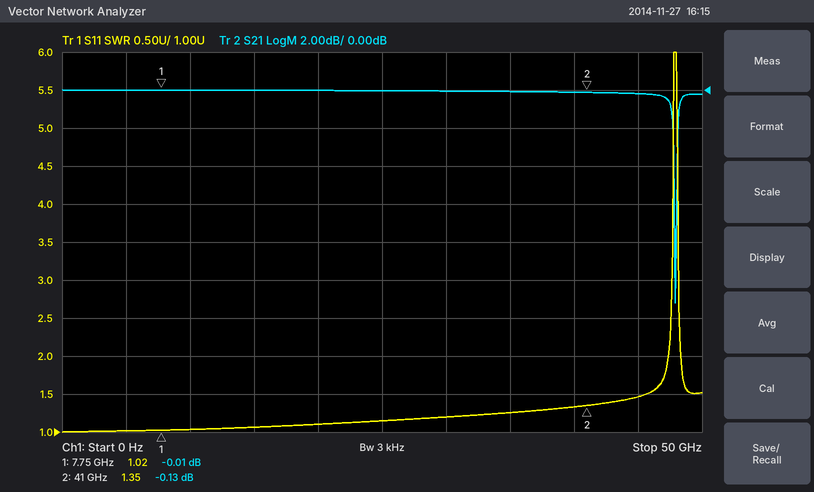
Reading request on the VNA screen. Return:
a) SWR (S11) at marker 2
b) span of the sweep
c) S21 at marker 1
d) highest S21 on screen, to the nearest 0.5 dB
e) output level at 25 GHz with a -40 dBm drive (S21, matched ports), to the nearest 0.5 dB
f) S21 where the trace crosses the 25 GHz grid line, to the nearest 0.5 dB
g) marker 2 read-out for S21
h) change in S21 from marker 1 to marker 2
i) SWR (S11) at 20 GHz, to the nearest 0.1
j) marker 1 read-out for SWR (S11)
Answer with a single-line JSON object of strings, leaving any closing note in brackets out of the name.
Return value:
{"SWR (S11) at marker 2": "1.35", "span of the sweep": "50 GHz", "S21 at marker 1": "-0.01 dB", "highest S21 on screen, to the nearest 0.5 dB": "0.0 dB", "output level at 25 GHz with a -40 dBm drive (S21, matched ports), to the nearest 0.5 dB": "-40.0 dBm", "S21 where the trace crosses the 25 GHz grid line, to the nearest 0.5 dB": "0.0 dB", "marker 2 read-out for S21": "-0.13 dB", "change in S21 from marker 1 to marker 2": "-0.12 dB", "SWR (S11) at 20 GHz, to the nearest 0.1": "1.1", "marker 1 read-out for SWR": "1.02"}
